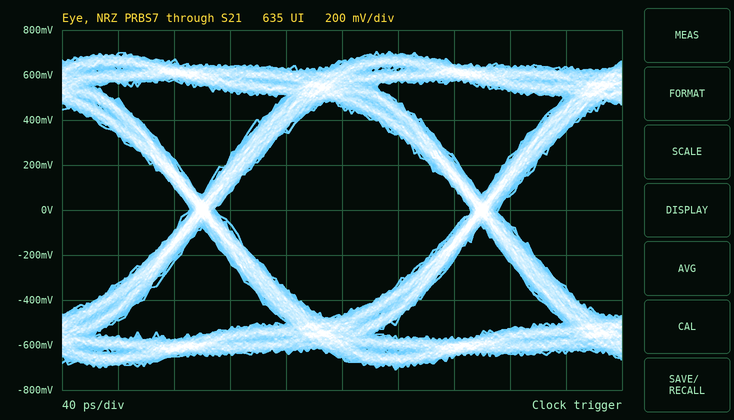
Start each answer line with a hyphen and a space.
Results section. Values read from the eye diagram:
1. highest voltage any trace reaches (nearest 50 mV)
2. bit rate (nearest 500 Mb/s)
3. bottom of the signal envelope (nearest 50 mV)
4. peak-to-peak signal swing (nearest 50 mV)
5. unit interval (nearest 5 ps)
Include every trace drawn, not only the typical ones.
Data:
- 700 mV
- 5.0 Gb/s
- -700 mV
- 1.40 V
- 200 ps
